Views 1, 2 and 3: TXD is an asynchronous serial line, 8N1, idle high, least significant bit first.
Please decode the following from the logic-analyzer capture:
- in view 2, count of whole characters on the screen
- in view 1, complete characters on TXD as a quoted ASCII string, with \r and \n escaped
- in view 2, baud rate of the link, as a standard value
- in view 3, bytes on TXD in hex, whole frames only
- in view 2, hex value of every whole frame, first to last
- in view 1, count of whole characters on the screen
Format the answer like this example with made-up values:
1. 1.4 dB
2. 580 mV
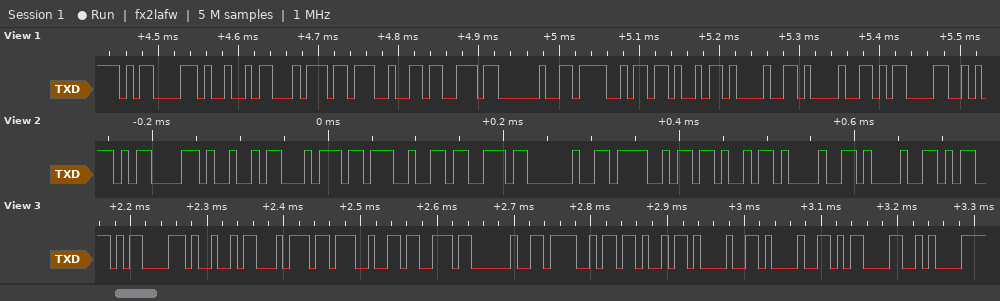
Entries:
1. 10
2. "\rIt's OK!!\r"
3. 115200 baud
4. 0D 49 74 27 73 20 4F 4B 21 21 0D 0A
5. 0x0D 0x49 0x74 0x27 0x73 0x20 0x4F 0x4B 0x21 0x21
6. 11
